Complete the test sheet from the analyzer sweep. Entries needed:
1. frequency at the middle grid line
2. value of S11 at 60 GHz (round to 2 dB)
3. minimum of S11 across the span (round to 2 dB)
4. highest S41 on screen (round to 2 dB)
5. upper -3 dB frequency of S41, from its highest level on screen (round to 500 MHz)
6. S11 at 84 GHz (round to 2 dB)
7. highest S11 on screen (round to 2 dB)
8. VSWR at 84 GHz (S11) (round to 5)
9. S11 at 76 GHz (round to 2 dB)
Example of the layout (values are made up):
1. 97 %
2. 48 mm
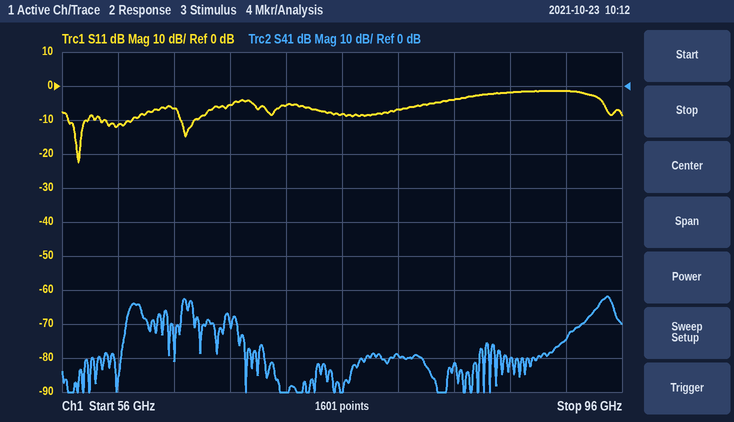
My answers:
1. 76 GHz
2. -12 dB
3. -22 dB
4. -62 dB
5. 95.5 GHz
6. -4 dB
7. -2 dB
8. 5
9. -8 dB
